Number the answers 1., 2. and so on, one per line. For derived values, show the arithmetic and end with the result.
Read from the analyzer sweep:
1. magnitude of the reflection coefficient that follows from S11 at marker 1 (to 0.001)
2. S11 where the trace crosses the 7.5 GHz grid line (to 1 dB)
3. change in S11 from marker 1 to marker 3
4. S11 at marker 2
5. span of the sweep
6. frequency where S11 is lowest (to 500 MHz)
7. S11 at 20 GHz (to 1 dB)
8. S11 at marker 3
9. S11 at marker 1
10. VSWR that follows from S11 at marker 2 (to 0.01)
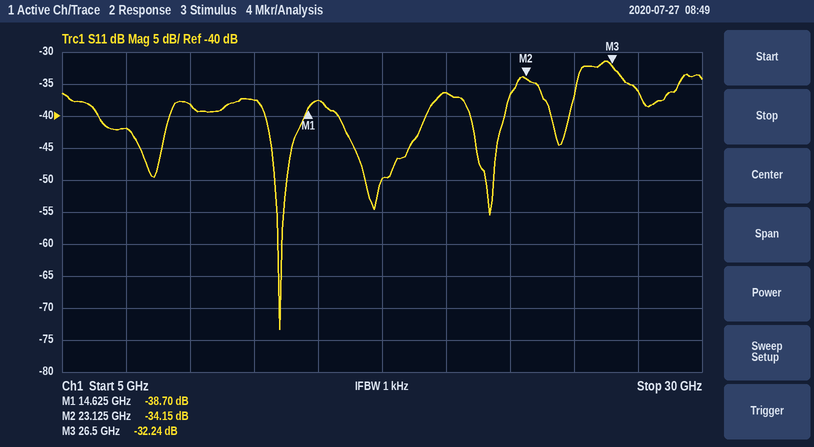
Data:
1. 10^(-38.7/20) ≈ 0.012
2. -42 dB
3. -32.24 − (-38.7) = 6.46 dB
4. -34.15 dB
5. 25 GHz
6. 13.5 GHz
7. -36 dB
8. -32.24 dB
9. -38.70 dB
10. (1 + 0.0196)/(1 − 0.0196) ≈ 1.04
